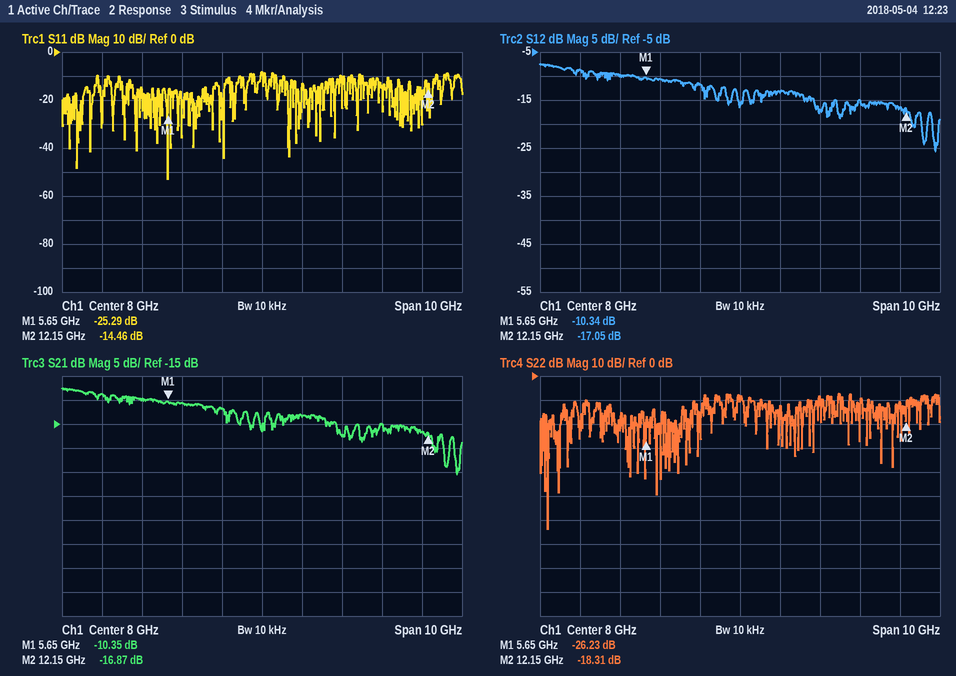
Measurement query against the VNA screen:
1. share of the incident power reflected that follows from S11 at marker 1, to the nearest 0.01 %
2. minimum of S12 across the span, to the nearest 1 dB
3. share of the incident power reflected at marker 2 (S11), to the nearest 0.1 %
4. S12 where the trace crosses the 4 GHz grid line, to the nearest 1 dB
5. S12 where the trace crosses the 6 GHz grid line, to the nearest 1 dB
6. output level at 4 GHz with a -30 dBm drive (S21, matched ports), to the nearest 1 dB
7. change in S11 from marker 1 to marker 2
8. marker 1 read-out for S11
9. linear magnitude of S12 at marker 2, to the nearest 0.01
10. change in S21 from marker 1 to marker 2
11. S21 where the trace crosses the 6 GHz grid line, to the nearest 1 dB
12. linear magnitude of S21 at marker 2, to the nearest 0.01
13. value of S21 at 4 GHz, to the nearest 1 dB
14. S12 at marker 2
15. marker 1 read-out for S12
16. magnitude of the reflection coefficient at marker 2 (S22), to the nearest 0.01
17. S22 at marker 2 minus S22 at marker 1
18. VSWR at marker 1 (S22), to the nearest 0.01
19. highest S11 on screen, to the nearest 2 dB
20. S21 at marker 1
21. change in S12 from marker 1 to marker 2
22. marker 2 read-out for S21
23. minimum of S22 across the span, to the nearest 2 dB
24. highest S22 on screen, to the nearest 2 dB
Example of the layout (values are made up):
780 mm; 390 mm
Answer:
0.30 %; -26 dB; 3.6 %; -9 dB; -11 dB; -39 dBm; 10.83 dB; -25.29 dB; 0.14; -6.52 dB; -11 dB; 0.14; -9 dB; -17.05 dB; -10.34 dB; 0.12; 7.92 dB; 1.10; -8 dB; -10.35 dB; -6.71 dB; -16.87 dB; -64 dB; -8 dB
